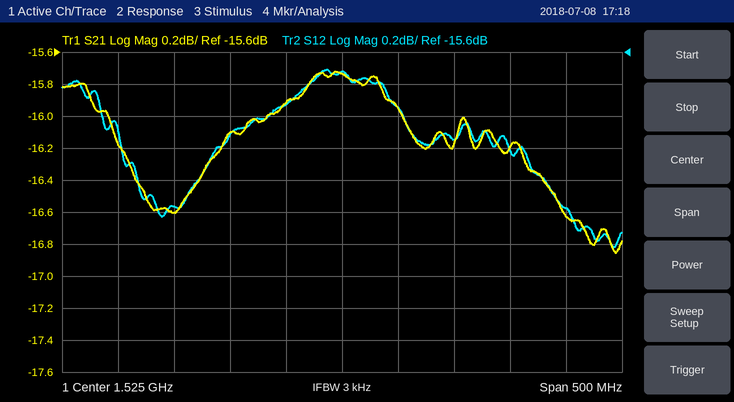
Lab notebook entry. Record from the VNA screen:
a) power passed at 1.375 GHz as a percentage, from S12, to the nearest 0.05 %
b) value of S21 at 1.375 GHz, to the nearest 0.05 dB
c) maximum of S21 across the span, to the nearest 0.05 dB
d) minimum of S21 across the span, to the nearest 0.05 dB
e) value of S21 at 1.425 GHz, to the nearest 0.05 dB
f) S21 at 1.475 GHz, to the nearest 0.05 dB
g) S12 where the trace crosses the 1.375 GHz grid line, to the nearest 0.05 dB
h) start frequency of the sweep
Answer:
2.20 %
-16.60 dB
-15.70 dB
-16.85 dB
-16.10 dB
-15.90 dB
-16.55 dB
1.275 GHz
